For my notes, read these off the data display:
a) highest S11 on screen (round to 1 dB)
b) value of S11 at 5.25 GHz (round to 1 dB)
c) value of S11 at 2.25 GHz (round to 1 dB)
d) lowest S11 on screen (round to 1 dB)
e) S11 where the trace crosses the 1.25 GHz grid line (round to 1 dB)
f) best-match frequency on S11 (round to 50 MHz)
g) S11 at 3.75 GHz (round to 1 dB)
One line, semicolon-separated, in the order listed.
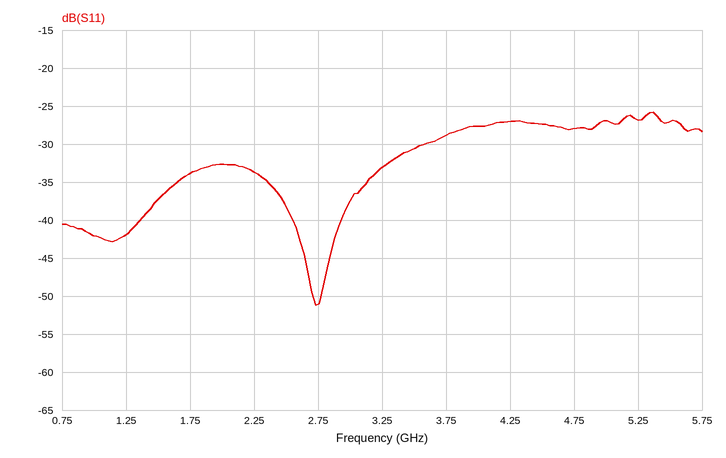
-26 dB; -27 dB; -34 dB; -51 dB; -42 dB; 2.75 GHz; -29 dB
